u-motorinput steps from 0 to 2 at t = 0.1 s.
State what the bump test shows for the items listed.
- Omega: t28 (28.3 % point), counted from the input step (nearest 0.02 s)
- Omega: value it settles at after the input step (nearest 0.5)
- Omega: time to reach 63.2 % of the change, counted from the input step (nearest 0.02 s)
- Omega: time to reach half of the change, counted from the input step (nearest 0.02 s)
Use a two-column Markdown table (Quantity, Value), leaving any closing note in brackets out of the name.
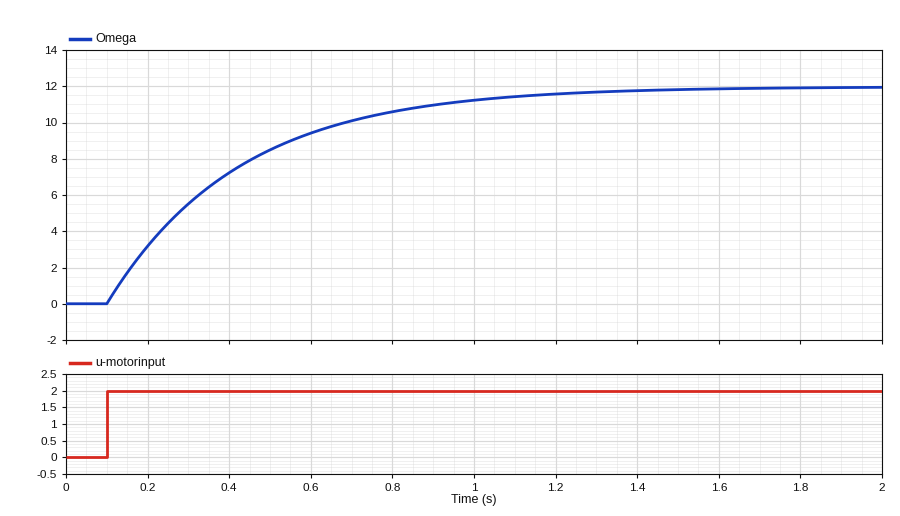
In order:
| Quantity | Value |
|---|---|
| Omega: t28 (28.3 % point), counted from the input step | 0.10 s |
| Omega: value it settles at after the input step | 12.0 |
| Omega: time to reach 63.2 % of the change, counted from the input step | 0.32 s |
| Omega: time to reach half of the change, counted from the input step | 0.22 s |
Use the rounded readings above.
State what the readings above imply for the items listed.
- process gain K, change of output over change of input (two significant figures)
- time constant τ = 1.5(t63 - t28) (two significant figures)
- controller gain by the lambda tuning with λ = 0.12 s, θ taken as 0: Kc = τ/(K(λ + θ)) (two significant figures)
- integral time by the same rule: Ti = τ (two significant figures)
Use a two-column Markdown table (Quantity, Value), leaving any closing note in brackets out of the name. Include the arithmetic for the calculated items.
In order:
| Quantity | Value |
|---|---|
| process gain K, change of output over change of input | (12 - 0) / 2 = 6.0 |
| time constant τ = 1.5(t63 - t28) | 1.5 × (0.32 - 0.1) = 0.33 s |
| controller gain by the lambda tuning with λ = 0.12 s, θ taken as 0: Kc = τ/(K(λ + θ)) | 0.33 / (6 × (0.12 + 0)) = 0.46 |
| integral time by the same rule: Ti = τ | 0.33 s |
